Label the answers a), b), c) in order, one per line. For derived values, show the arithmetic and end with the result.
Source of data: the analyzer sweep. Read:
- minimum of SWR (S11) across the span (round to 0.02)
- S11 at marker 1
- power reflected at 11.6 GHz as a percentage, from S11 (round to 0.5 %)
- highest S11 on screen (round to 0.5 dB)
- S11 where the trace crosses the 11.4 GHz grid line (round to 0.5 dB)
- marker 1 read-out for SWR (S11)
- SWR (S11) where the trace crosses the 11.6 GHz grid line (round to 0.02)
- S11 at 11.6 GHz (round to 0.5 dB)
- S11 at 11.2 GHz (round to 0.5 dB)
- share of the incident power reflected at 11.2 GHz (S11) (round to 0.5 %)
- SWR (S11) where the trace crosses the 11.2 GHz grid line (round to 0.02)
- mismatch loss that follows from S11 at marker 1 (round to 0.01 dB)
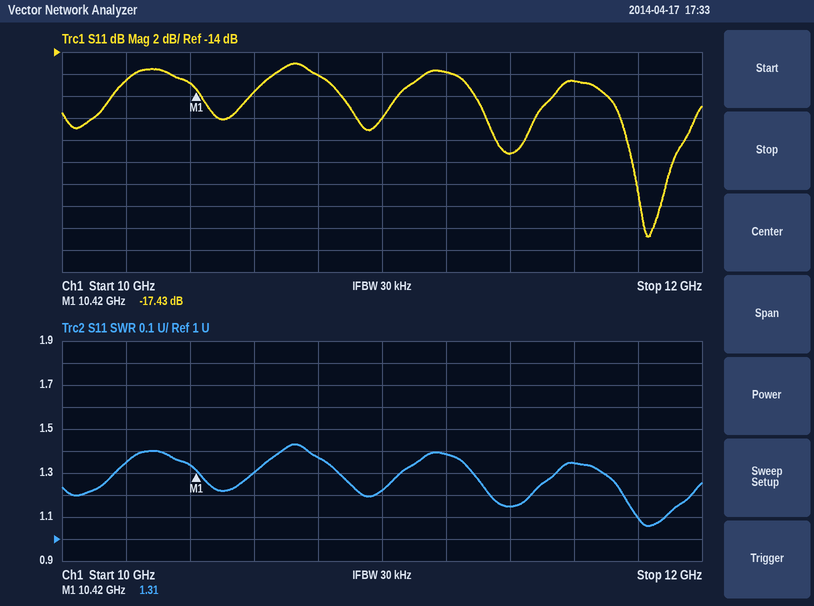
a) 1.06
b) -17.43 dB
c) 10^(-16.5/10) ≈ 2.24 %, so 2.0 % to the nearest 0.5 %
d) -15.0 dB
e) -23.0 dB
f) 1.31
g) 1.34
h) -16.5 dB
i) -16.0 dB
j) 10^(-16/10) ≈ 2.5 %
k) 1.38
l) −10 log10(1 − 10^(-17.43/10)) ≈ 0.08 dB
